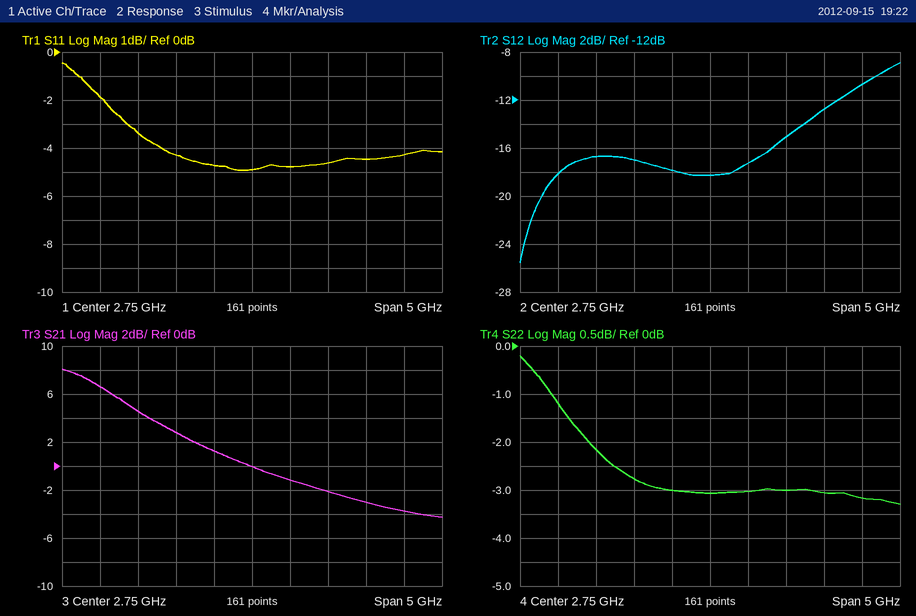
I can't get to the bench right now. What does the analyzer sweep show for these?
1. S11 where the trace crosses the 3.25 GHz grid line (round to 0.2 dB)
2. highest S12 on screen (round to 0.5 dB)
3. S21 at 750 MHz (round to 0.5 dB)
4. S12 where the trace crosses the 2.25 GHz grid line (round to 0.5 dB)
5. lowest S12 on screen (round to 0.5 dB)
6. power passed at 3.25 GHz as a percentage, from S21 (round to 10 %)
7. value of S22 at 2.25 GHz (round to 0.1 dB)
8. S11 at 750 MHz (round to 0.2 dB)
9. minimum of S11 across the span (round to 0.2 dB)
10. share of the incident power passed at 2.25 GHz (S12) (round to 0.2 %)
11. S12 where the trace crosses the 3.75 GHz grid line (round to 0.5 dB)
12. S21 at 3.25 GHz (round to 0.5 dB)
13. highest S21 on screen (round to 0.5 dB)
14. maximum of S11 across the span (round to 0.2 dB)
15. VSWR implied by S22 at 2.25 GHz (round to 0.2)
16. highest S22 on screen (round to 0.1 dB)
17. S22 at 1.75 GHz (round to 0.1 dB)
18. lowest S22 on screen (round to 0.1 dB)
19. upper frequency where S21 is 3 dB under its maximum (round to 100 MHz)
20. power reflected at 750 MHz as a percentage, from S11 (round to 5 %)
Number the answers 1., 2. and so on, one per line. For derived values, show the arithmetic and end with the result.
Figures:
1. -4.8 dB
2. -9.0 dB
3. 6.5 dB
4. -18.0 dB
5. -25.5 dB
6. 10^(-1/10) ≈ 79.4 %, so 80 % to the nearest 10 %
7. -3.0 dB
8. -1.8 dB
9. -5.0 dB
10. 10^(-18/10) ≈ 1.6 %
11. -15.0 dB
12. -1.0 dB
13. 8.0 dB
14. -0.4 dB
15. |Γ| = 10^(-3/20) = 0.7079; VSWR = (1 + 0.7079)/(1 − 0.7079) ≈ 5.8
16. -0.2 dB
17. -2.8 dB
18. -3.3 dB
19. 1.1 GHz
20. 10^(-1.8/10) ≈ 66.1 %, so 65 % to the nearest 5 %
